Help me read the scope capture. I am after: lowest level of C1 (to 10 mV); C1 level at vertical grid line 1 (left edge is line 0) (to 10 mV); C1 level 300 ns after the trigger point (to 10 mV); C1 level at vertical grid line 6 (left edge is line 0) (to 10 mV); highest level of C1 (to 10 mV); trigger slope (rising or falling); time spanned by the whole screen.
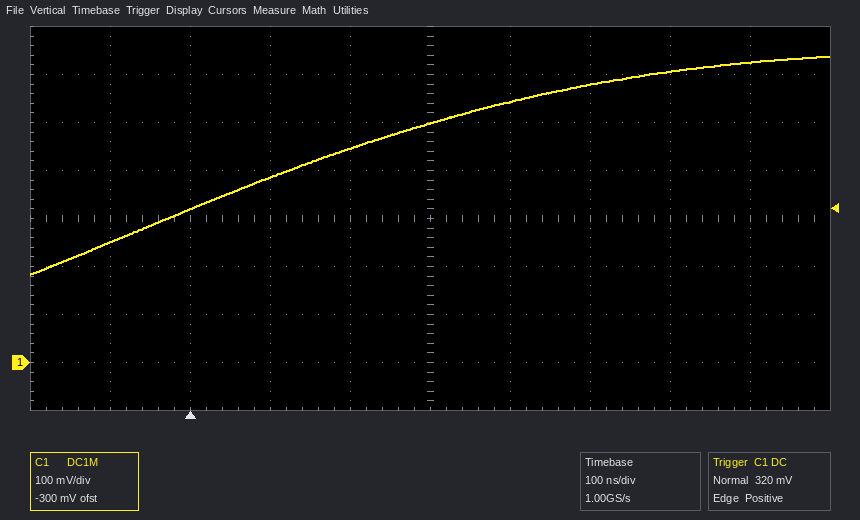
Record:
180 mV
250 mV
500 mV
540 mV
640 mV
rising
1 µs
